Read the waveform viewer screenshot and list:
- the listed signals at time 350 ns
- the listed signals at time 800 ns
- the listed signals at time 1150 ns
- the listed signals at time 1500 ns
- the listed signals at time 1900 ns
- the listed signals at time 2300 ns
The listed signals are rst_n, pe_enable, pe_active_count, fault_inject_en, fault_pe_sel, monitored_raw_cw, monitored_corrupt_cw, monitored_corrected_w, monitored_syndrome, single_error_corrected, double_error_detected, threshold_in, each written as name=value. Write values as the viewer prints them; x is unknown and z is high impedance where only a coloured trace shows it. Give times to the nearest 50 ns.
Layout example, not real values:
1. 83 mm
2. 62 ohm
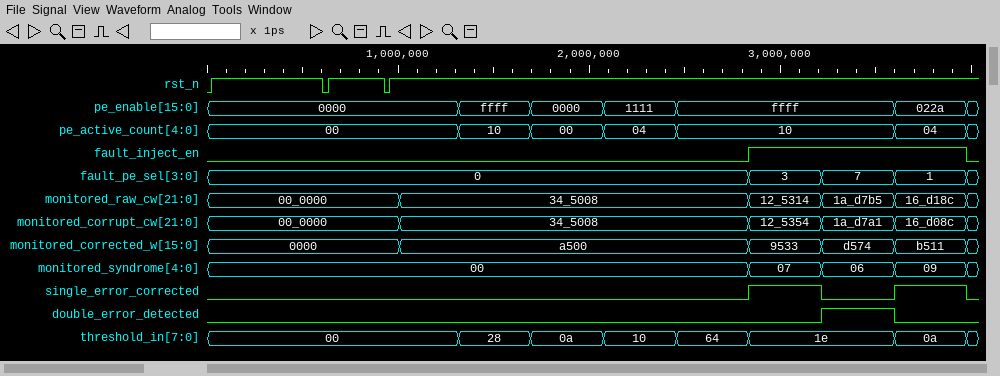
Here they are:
1. rst_n=1, pe_enable=0000, pe_active_count=00, fault_inject_en=0, fault_pe_sel=0, monitored_raw_cw=00_0000, monitored_corrupt_cw=00_0000, monitored_corrected_w=0000, monitored_syndrome=00, single_error_corrected=0, double_error_detected=0, threshold_in=00
2. rst_n=1, pe_enable=0000, pe_active_count=00, fault_inject_en=0, fault_pe_sel=0, monitored_raw_cw=00_0000, monitored_corrupt_cw=00_0000, monitored_corrected_w=0000, monitored_syndrome=00, single_error_corrected=0, double_error_detected=0, threshold_in=00
3. rst_n=1, pe_enable=0000, pe_active_count=00, fault_inject_en=0, fault_pe_sel=0, monitored_raw_cw=34_5008, monitored_corrupt_cw=34_5008, monitored_corrected_w=a500, monitored_syndrome=00, single_error_corrected=0, double_error_detected=0, threshold_in=00
4. rst_n=1, pe_enable=ffff, pe_active_count=10, fault_inject_en=0, fault_pe_sel=0, monitored_raw_cw=34_5008, monitored_corrupt_cw=34_5008, monitored_corrected_w=a500, monitored_syndrome=00, single_error_corrected=0, double_error_detected=0, threshold_in=28
5. rst_n=1, pe_enable=0000, pe_active_count=00, fault_inject_en=0, fault_pe_sel=0, monitored_raw_cw=34_5008, monitored_corrupt_cw=34_5008, monitored_corrected_w=a500, monitored_syndrome=00, single_error_corrected=0, double_error_detected=0, threshold_in=0a
6. rst_n=1, pe_enable=1111, pe_active_count=04, fault_inject_en=0, fault_pe_sel=0, monitored_raw_cw=34_5008, monitored_corrupt_cw=34_5008, monitored_corrected_w=a500, monitored_syndrome=00, single_error_corrected=0, double_error_detected=0, threshold_in=10
